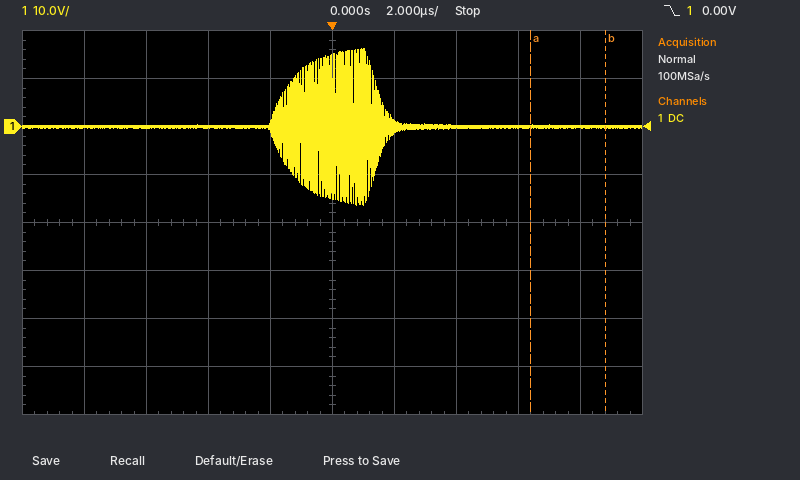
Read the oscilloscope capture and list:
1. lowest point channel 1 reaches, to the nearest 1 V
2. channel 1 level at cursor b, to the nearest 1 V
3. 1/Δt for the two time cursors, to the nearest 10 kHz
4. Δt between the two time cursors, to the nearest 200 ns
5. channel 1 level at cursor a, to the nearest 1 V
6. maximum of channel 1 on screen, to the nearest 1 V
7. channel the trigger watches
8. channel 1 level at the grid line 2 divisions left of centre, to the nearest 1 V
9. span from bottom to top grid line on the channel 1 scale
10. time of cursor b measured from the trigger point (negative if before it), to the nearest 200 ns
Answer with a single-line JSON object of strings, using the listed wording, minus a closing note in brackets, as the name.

{"lowest point channel 1 reaches, to the nearest 1 V": "-16 V", "channel 1 level at cursor b, to the nearest 1 V": "0 V", "1/Δt for the two time cursors, to the nearest 10 kHz": "420 kHz", "Δt between the two time cursors, to the nearest 200 ns": "2.4 µs", "channel 1 level at cursor a, to the nearest 1 V": "0 V", "maximum of channel 1 on screen, to the nearest 1 V": "16 V", "channel the trigger watches": "channel 1", "channel 1 level at the grid line 2 divisions left of centre, to the nearest 1 V": "0 V", "span from bottom to top grid line on the channel 1 scale": "80 V", "time of cursor b measured from the trigger point (negative if before it), to the nearest 200 ns": "+8.8 µs"}
